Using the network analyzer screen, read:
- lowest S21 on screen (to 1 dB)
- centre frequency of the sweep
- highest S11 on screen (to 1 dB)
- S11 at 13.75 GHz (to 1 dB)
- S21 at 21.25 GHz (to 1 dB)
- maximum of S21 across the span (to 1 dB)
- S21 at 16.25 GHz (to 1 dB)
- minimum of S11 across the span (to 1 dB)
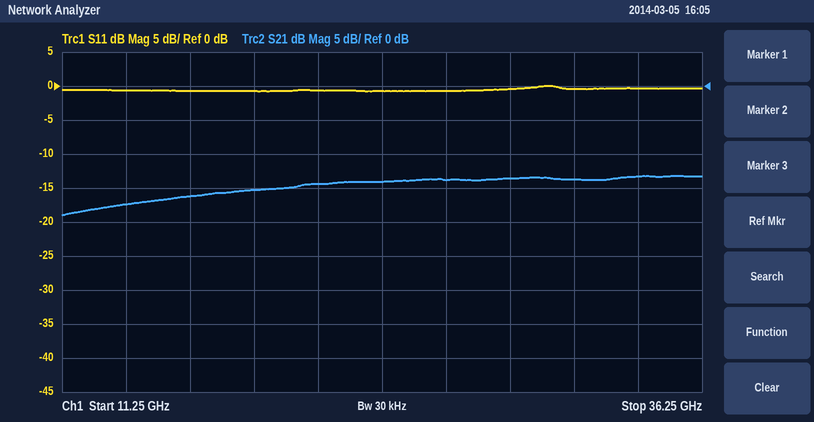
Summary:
-19 dB
23.75 GHz
0 dB
-1 dB
-14 dB
-13 dB
-16 dB
-1 dB
